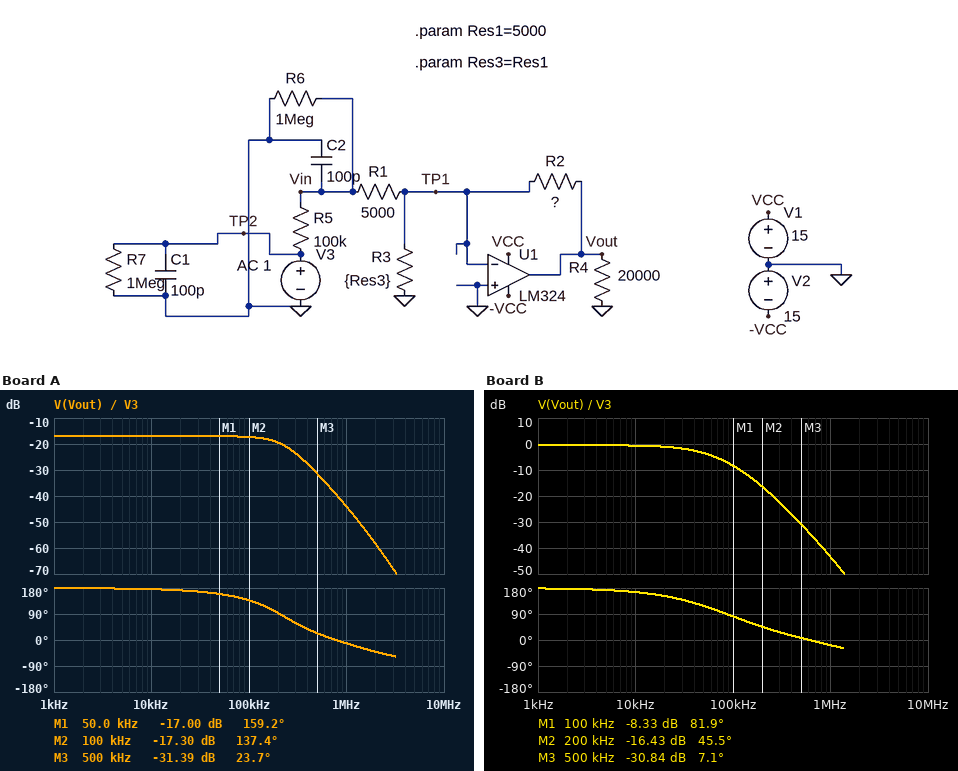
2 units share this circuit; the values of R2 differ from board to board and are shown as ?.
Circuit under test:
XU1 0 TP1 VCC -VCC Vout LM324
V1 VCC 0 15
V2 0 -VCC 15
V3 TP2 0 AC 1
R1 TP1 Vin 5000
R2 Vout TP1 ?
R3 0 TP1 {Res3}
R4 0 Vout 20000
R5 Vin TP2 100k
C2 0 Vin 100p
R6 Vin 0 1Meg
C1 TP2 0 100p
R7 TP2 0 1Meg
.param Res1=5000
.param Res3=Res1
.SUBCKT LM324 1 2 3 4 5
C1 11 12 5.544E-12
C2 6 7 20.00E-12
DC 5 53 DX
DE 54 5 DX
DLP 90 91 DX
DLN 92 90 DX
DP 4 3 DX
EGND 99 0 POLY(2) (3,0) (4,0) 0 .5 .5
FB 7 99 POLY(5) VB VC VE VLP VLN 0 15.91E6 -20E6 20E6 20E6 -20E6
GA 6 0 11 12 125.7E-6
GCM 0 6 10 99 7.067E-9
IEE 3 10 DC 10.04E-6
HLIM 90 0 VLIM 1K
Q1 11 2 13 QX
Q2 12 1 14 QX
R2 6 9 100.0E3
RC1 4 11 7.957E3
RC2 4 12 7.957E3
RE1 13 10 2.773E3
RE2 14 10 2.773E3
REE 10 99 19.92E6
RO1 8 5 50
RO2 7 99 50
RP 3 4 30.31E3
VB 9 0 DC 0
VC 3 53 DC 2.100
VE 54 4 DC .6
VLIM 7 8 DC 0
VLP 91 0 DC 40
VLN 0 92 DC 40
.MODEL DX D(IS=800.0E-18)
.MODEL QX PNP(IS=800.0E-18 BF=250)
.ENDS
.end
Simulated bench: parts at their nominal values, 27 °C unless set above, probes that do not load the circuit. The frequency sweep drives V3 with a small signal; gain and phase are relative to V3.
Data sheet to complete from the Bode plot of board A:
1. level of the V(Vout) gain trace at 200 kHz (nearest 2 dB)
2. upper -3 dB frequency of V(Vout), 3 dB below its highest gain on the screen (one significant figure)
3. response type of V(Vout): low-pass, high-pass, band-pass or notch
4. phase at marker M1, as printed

-20 dB
200 kHz
low-pass
159.2 deg
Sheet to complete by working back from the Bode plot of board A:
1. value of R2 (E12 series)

15 kΩ
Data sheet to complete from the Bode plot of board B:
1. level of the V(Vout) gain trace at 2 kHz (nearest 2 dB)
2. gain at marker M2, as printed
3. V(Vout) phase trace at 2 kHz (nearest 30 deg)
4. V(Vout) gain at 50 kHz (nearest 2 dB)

0 dB
-16.43 dB
180 deg
-4 dB
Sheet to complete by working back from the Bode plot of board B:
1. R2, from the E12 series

100 kΩ
